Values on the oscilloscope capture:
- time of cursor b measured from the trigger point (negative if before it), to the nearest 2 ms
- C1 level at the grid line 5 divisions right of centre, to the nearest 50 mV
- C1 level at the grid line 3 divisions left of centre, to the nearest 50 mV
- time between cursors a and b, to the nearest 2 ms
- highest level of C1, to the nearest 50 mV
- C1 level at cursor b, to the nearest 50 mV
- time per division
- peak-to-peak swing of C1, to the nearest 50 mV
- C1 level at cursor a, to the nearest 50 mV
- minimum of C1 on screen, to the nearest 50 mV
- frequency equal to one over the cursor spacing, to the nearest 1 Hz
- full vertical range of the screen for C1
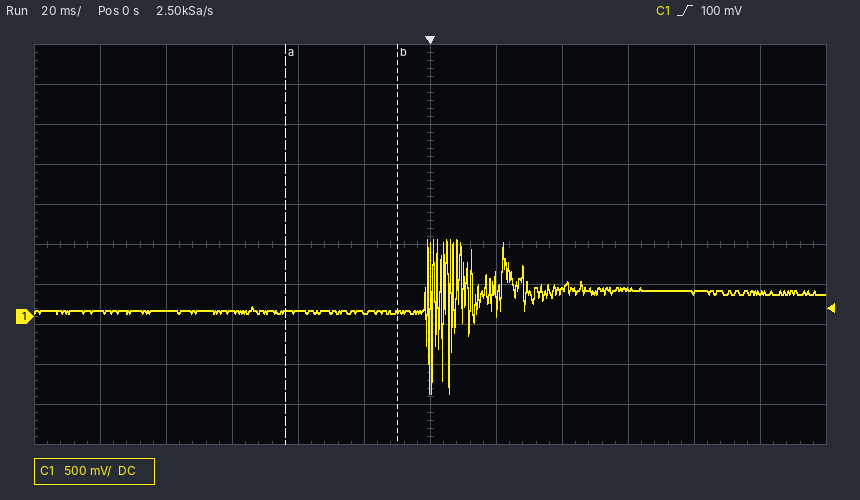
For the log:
-10 ms
300 mV
50 mV
34 ms
950 mV
50 mV
20 ms
1.90 V
50 mV
-950 mV
29 Hz
5 V
